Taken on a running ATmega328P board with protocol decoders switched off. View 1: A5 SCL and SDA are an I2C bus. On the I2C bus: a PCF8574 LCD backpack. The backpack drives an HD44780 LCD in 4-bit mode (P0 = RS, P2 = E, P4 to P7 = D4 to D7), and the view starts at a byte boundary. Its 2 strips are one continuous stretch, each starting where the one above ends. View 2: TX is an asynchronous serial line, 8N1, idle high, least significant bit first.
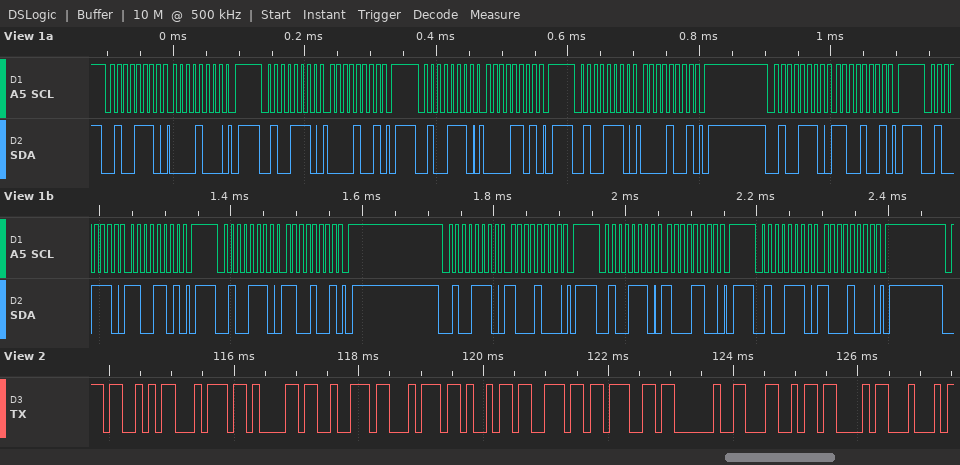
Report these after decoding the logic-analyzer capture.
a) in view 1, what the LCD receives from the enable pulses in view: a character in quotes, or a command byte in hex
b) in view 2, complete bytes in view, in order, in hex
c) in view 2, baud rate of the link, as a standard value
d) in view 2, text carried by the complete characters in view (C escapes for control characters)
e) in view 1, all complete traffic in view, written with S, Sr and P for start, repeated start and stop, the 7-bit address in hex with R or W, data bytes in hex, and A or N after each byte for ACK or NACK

data 0x0C
53 74 61 72 74 69 6E 67 20 4C 43 44
9600 baud
"Starting LCD"
S 27W A 08 A P S 27W A 09 A P S 27W A 0D A P S 27W A 09 A P S 27W A C9 A P S 27W A CD A P S 27W A C9 A P S 27W A 88 A P S 27W A 8C A P S 27W A 88 A P
